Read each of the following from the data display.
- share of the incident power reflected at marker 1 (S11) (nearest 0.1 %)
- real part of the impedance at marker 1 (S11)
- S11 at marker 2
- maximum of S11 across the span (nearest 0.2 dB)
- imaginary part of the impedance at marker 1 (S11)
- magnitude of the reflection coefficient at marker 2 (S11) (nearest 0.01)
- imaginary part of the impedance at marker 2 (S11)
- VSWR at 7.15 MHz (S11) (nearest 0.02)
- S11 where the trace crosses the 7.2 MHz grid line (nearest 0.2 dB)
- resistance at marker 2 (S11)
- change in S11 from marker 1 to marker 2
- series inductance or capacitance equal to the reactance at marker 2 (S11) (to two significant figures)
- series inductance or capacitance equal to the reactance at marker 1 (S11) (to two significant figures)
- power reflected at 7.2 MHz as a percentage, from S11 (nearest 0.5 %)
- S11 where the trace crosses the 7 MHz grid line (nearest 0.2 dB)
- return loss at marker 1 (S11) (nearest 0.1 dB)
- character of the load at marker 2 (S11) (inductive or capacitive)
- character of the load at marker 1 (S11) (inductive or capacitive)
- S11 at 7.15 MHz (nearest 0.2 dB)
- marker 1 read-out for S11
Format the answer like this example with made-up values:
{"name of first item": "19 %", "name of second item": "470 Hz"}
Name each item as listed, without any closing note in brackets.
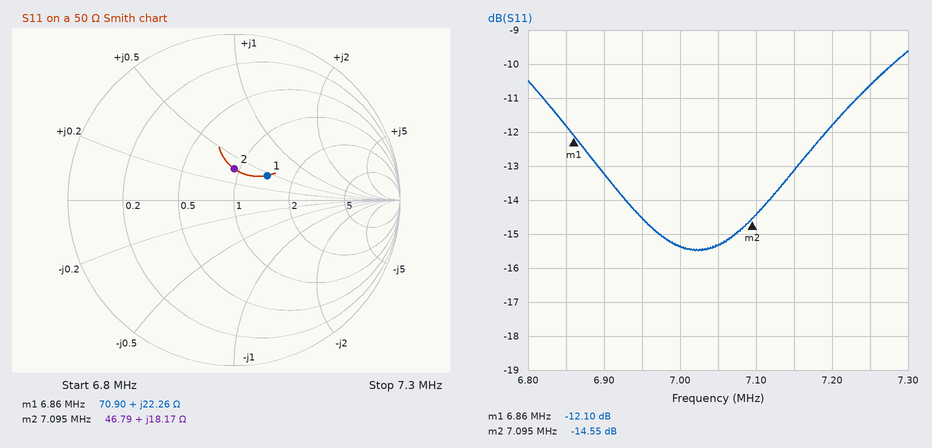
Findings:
{"share of the incident power reflected at marker 1 (S11)": "6.2 %", "real part of the impedance at marker 1": "70.90 Ω", "S11 at marker 2": "-14.55 dB", "maximum of S11 across the span": "-9.6 dB", "imaginary part of the impedance at marker 1": "+22.26 Ω", "magnitude of the reflection coefficient at marker 2 (S11)": "0.19", "imaginary part of the impedance at marker 2": "+18.17 Ω", "VSWR at 7.15 MHz (S11)": "1.56", "S11 where the trace crosses the 7.2 MHz grid line": "-11.8 dB", "resistance at marker 2": "46.79 Ω", "change in S11 from marker 1 to marker 2": "-2.45 dB", "series inductance or capacitance equal to the reactance at marker 2 (S11)": "410 nH", "series inductance or capacitance equal to the reactance at marker 1 (S11)": "520 nH", "power reflected at 7.2 MHz as a percentage, from S11": "6.5 %", "S11 where the trace crosses the 7 MHz grid line": "-15.4 dB", "return loss at marker 1 (S11)": "12.1 dB", "character of the load at marker 2 (S11)": "inductive", "character of the load at marker 1 (S11)": "inductive", "S11 at 7.15 MHz": "-13.2 dB", "marker 1 read-out for S11": "-12.10 dB"}
